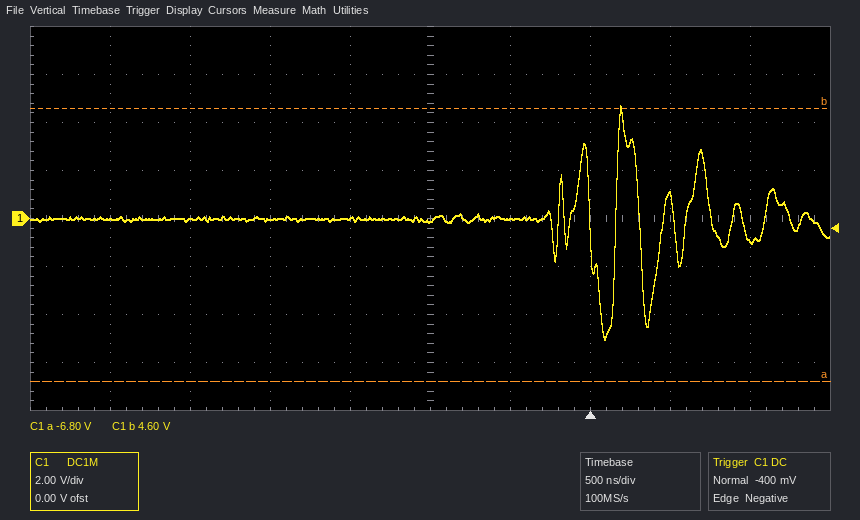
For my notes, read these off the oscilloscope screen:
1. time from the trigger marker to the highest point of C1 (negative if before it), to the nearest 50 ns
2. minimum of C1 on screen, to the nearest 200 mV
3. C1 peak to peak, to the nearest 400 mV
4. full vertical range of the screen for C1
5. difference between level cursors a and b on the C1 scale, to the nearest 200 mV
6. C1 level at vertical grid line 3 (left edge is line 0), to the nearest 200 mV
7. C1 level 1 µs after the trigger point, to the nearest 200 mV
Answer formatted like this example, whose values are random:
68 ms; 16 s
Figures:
+200 ns; -5.0 V; 9.6 V; 16 V; 11.4 V; 0.0 V; -800 mV
